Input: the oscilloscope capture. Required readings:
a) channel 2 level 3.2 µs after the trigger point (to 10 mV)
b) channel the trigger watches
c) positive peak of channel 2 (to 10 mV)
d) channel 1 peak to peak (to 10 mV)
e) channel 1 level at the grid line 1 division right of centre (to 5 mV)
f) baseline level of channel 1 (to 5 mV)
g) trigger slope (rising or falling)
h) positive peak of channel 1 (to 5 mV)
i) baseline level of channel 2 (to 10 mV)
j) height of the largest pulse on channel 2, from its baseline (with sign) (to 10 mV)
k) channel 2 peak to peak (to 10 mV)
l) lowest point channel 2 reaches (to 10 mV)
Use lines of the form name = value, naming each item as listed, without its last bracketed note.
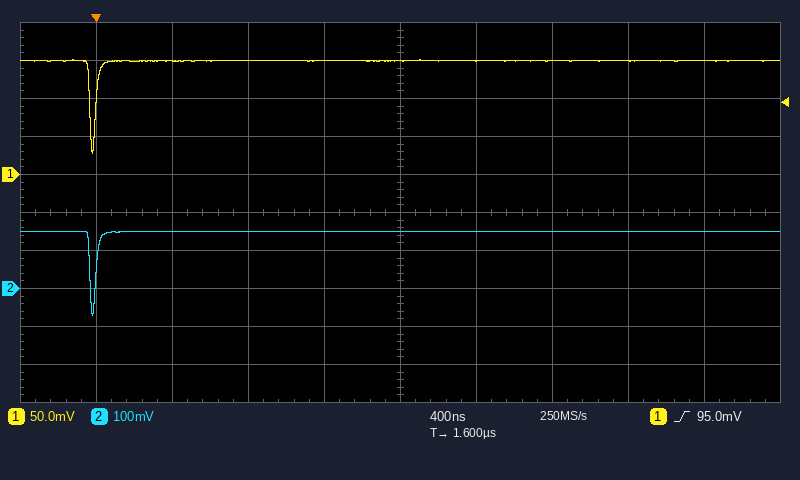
channel 2 level 3.2 µs after the trigger point = 150 mV
channel the trigger watches = channel 1
positive peak of channel 2 = 150 mV
channel 1 peak to peak = 120 mV
channel 1 level at the grid line 1 division right of centre = 150 mV
baseline level of channel 1 = 150 mV
trigger slope = rising
positive peak of channel 1 = 150 mV
baseline level of channel 2 = 150 mV
height of the largest pulse on channel 2, from its baseline (with sign) = -220 mV
channel 2 peak to peak = 220 mV
lowest point channel 2 reaches = -70 mV
